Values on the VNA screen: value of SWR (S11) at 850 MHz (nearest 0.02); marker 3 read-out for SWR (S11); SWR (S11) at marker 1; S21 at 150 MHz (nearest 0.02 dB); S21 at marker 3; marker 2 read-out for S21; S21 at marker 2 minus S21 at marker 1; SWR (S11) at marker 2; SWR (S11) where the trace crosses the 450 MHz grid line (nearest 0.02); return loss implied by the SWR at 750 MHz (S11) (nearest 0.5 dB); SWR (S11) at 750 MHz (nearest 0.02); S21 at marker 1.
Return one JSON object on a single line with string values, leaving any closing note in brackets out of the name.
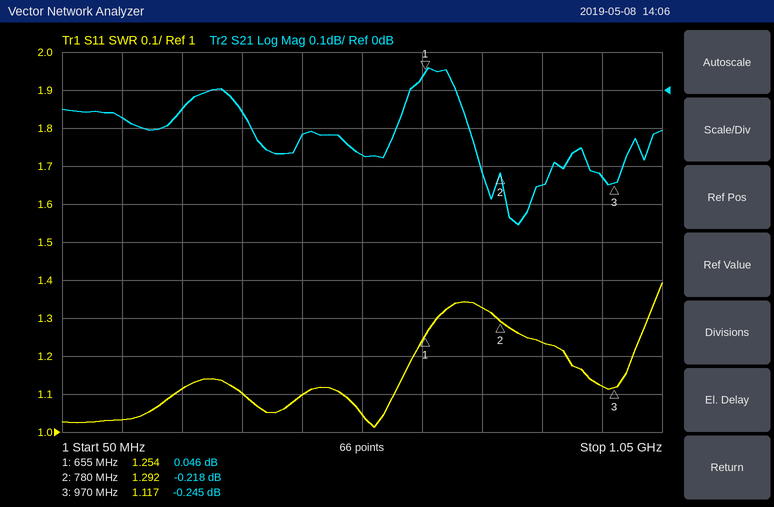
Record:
{"value of SWR (S11) at 850 MHz": "1.24", "marker 3 read-out for SWR": "1.117", "SWR (S11) at marker 1": "1.254", "S21 at 150 MHz": "-0.08 dB", "S21 at marker 3": "-0.245 dB", "marker 2 read-out for S21": "-0.218 dB", "S21 at marker 2 minus S21 at marker 1": "-0.264 dB", "SWR (S11) at marker 2": "1.292", "SWR (S11) where the trace crosses the 450 MHz grid line": "1.10", "return loss implied by the SWR at 750 MHz (S11)": "17.0 dB", "SWR (S11) at 750 MHz": "1.32", "S21 at marker 1": "0.046 dB"}
